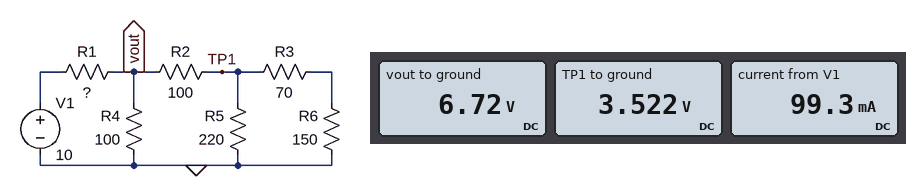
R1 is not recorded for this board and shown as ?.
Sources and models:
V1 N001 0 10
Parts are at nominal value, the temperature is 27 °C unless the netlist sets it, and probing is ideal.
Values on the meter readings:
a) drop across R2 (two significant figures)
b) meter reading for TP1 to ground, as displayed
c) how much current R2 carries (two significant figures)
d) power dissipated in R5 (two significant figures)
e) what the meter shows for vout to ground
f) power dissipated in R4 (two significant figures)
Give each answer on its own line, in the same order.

3.2 V
3.522 V
32 mA
56 mW
6.72 V
450 mW
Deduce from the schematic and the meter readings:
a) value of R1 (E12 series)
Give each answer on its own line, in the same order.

33 Ω
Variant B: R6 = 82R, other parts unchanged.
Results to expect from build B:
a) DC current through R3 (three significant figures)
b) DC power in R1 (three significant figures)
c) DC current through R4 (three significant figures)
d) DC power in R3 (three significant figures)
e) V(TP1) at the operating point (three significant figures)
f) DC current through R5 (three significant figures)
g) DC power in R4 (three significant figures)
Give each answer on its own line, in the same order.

20.7 mA
340 mW
66.5 mA
30.0 mW
3.15 V
14.3 mA
442 mW
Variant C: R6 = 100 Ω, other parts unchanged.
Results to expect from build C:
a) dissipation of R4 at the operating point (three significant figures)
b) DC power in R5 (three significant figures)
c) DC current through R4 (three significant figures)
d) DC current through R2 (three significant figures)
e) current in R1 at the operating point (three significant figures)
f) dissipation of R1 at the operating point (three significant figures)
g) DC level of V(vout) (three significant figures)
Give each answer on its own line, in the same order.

445 mW
48.5 mW
66.7 mA
34.1 mA
101 mA
335 mW
6.67 V
